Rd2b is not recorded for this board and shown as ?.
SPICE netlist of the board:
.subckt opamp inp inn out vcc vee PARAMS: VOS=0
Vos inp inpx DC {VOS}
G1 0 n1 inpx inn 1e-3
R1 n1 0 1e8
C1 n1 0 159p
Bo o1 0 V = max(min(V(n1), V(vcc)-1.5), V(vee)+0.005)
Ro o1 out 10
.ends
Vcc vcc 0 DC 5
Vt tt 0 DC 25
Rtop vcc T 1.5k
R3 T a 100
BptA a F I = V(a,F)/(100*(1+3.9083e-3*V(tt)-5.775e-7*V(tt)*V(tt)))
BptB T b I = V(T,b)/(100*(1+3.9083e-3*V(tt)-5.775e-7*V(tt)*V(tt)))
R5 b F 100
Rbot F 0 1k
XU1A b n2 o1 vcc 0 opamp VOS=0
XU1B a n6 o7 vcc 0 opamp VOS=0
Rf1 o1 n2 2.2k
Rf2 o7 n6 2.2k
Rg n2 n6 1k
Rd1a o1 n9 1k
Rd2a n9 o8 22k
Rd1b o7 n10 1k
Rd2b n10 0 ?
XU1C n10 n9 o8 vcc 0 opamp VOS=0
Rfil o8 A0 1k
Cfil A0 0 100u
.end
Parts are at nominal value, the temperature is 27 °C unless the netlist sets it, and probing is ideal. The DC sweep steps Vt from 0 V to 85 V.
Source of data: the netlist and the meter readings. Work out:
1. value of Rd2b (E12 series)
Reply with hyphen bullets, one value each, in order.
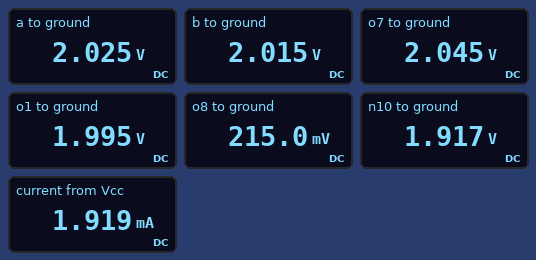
- 15 kΩ
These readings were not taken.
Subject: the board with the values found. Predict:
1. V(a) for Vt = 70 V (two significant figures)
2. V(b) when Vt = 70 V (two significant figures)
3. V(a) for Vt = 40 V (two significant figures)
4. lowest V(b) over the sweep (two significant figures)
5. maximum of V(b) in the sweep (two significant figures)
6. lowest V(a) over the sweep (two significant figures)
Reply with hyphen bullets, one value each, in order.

- 2.0 V
- 2.0 V
- 2.0 V
- 2.0 V
- 2.0 V
- 2.0 V
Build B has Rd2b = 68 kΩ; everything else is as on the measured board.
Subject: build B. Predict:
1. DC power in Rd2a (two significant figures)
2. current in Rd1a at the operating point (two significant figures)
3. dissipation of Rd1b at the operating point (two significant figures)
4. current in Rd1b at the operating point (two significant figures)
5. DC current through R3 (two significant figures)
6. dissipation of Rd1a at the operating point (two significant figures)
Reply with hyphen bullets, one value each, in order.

- 9.5 µW
- 21 µA
- 880 nW
- 30 µA
- 960 µA
- 430 nW
